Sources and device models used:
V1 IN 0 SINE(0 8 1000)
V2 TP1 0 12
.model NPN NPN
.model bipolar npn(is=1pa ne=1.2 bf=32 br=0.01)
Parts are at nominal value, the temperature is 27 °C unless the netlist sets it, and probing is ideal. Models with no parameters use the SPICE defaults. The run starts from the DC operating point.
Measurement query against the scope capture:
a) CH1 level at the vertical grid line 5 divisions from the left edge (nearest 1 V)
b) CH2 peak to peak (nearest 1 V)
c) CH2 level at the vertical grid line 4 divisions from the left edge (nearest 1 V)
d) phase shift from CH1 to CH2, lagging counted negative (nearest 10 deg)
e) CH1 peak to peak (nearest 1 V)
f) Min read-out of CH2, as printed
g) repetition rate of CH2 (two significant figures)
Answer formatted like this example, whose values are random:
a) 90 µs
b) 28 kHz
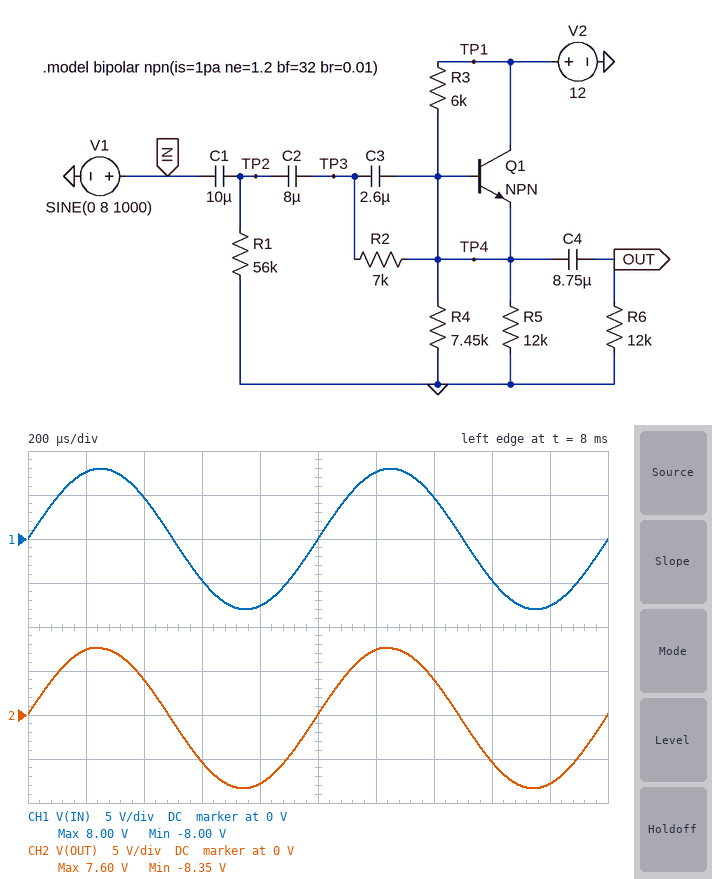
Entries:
a) 0 V
b) 16 V
c) -8 V
d) 0 deg
e) 16 V
f) -8.35 V
g) 1.0 kHz
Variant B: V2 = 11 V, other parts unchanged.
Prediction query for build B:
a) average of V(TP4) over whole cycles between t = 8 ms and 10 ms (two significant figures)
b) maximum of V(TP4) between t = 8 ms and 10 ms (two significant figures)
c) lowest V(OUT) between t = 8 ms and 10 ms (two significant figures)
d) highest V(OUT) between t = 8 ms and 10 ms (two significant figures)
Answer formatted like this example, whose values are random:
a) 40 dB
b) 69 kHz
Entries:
a) 3.9 V
b) 12 V
c) -8.8 V
d) 7.1 V
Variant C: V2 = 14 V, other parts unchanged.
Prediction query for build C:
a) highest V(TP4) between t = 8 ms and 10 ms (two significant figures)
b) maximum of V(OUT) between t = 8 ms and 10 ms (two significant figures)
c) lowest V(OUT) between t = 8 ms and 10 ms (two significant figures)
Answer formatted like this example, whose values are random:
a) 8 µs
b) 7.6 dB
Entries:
a) 14 V
b) 8.0 V
c) -8.0 V
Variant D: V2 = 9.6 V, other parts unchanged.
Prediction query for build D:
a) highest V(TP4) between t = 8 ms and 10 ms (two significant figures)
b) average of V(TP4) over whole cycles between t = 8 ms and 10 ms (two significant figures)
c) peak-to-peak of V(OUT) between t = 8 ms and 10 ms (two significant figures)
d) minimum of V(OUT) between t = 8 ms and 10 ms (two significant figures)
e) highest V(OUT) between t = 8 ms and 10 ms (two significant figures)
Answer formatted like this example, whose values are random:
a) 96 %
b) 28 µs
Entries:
a) 10 V
b) 2.6 V
c) 16 V
d) -9.4 V
e) 6.4 V
